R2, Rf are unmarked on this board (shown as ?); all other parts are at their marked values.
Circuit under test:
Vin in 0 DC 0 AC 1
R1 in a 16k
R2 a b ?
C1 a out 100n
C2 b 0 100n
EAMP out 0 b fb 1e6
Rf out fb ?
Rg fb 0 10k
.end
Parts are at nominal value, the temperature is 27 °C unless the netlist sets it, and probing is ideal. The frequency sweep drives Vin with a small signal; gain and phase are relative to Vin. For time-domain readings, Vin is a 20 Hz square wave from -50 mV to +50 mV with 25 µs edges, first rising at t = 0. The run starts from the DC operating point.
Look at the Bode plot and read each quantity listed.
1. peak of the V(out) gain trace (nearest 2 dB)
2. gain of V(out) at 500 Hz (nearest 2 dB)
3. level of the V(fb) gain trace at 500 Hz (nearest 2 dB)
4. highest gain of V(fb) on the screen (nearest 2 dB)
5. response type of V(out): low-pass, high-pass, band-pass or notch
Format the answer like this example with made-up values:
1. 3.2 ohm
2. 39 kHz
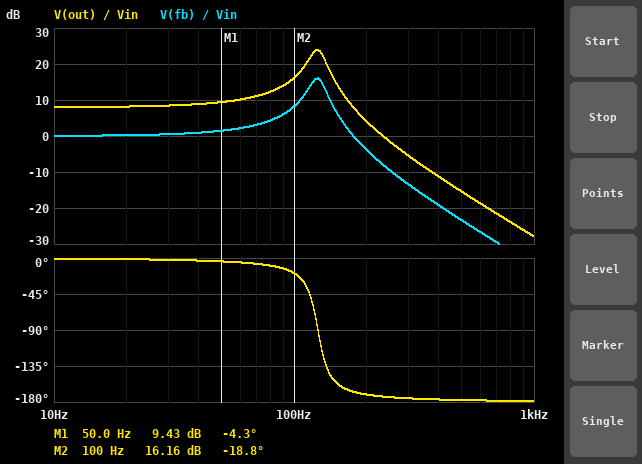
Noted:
1. 24 dB
2. -16 dB
3. -24 dB
4. 16 dB
5. low-pass
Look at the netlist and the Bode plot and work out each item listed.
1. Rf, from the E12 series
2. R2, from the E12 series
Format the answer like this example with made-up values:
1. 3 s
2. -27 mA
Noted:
1. 15 kΩ
2. 10 kΩ
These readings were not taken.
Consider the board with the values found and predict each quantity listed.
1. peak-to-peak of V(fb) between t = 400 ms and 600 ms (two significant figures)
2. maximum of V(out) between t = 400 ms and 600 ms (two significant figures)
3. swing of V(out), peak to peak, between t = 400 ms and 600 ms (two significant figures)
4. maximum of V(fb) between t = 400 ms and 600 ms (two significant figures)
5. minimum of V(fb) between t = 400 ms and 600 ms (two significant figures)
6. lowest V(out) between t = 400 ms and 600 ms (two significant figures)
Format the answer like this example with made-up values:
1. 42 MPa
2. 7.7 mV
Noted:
1. 230 mV
2. 290 mV
3. 580 mV
4. 120 mV
5. -120 mV
6. -290 mV
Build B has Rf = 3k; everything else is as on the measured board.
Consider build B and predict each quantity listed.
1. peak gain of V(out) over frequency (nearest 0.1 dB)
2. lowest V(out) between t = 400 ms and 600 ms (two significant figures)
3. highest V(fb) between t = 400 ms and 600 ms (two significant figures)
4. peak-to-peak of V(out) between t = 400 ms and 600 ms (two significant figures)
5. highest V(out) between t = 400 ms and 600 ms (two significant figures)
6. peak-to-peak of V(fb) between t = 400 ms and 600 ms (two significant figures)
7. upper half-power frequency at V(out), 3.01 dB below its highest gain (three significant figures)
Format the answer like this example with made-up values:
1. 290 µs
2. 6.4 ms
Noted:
1. 2.3 dB
2. -66 mV
3. 51 mV
4. 130 mV
5. 66 mV
6. 100 mV
7. 103 Hz
